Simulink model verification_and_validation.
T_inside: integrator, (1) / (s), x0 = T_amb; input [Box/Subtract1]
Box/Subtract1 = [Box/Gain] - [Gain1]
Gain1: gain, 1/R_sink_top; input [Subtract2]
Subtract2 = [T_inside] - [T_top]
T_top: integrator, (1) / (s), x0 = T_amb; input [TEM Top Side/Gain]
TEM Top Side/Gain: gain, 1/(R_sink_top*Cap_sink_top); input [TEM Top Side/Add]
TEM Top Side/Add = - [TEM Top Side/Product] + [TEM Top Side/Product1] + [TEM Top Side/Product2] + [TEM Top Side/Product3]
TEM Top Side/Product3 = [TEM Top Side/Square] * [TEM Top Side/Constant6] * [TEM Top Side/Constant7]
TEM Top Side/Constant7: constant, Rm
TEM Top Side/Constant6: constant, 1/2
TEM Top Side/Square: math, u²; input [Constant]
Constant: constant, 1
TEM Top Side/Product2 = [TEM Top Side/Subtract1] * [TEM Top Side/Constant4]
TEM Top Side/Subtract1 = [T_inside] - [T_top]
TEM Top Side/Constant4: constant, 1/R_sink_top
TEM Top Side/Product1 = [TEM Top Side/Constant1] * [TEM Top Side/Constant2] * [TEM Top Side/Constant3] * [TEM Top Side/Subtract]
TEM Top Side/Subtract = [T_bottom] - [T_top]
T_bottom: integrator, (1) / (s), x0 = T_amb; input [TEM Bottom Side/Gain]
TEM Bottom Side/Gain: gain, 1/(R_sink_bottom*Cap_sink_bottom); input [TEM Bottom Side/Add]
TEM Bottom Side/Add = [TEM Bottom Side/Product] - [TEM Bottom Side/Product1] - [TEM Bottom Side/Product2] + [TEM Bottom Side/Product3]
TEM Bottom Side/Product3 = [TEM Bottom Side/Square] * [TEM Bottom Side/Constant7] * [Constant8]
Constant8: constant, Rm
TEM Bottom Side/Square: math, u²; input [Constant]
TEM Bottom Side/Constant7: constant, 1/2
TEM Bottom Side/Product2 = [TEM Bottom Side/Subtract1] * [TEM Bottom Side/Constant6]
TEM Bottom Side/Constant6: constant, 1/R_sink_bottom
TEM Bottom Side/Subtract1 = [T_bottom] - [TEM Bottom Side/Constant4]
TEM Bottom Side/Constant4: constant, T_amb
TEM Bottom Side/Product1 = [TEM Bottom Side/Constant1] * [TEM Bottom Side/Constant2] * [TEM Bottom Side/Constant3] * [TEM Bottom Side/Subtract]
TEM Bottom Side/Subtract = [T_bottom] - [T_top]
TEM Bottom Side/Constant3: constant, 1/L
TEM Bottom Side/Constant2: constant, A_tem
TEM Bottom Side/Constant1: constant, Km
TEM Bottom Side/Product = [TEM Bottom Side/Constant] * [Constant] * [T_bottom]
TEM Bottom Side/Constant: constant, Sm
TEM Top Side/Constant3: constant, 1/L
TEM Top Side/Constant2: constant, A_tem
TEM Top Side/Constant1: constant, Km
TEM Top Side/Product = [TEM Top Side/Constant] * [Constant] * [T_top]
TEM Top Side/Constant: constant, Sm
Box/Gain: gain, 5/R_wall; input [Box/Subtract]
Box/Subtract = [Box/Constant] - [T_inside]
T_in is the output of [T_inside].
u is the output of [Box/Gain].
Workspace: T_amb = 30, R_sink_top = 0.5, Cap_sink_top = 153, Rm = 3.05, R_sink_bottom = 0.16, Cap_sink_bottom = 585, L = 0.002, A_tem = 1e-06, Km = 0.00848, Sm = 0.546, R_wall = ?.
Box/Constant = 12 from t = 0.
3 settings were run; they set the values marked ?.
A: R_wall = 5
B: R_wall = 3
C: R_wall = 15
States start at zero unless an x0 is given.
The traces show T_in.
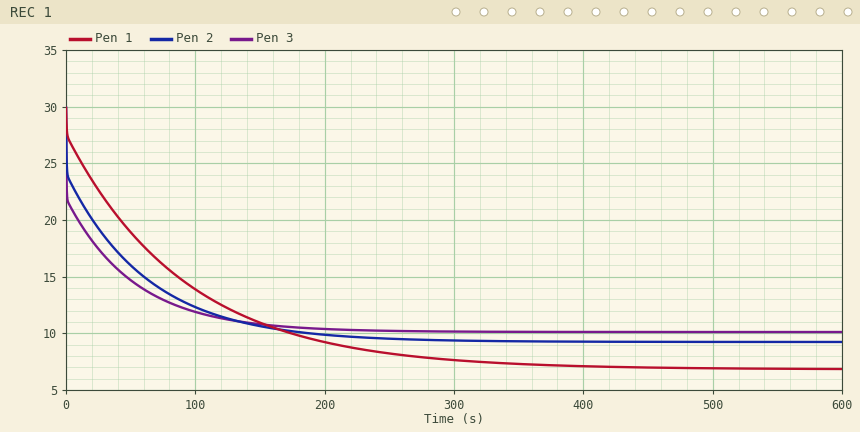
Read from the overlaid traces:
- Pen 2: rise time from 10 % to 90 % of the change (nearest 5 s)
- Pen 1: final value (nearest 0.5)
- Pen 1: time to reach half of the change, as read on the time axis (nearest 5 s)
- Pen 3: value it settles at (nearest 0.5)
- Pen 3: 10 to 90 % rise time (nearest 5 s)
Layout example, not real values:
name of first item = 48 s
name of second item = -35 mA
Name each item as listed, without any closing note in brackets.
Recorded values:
Pen 2: rise time from 10 % to 90 % of the change = 125 s
Pen 1: final value = 7.0
Pen 1: time to reach half of the change, as read on the time axis = 55 s
Pen 3: value it settles at = 10.0
Pen 3: 10 to 90 % rise time = 95 s
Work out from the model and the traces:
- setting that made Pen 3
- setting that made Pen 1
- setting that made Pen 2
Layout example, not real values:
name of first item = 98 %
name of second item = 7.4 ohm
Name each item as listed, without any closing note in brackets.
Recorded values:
setting that made Pen 3 = B
setting that made Pen 1 = C
setting that made Pen 2 = A
